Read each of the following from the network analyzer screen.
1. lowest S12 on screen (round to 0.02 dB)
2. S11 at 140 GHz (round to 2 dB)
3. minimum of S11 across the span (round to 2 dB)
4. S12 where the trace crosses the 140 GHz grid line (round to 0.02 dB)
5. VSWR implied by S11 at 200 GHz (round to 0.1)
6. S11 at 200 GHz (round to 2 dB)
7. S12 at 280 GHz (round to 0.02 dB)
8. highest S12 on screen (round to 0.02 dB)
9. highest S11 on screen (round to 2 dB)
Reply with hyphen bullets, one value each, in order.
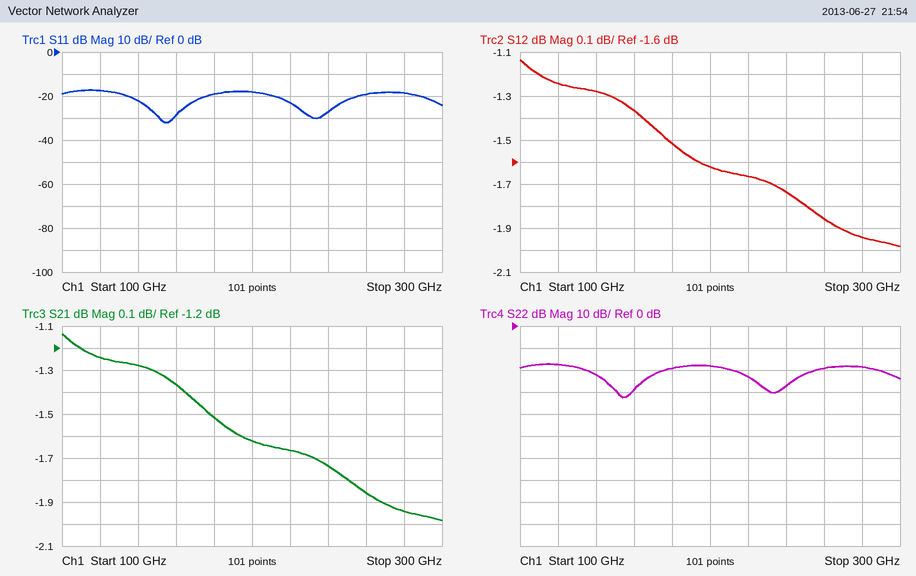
- -1.98 dB
- -22 dB
- -32 dB
- -1.28 dB
- 1.3
- -18 dB
- -1.94 dB
- -1.14 dB
- -18 dB
